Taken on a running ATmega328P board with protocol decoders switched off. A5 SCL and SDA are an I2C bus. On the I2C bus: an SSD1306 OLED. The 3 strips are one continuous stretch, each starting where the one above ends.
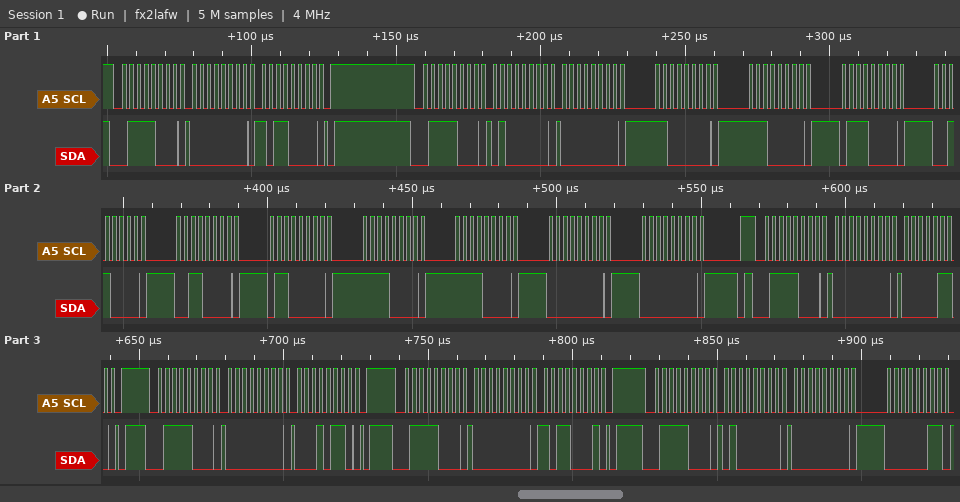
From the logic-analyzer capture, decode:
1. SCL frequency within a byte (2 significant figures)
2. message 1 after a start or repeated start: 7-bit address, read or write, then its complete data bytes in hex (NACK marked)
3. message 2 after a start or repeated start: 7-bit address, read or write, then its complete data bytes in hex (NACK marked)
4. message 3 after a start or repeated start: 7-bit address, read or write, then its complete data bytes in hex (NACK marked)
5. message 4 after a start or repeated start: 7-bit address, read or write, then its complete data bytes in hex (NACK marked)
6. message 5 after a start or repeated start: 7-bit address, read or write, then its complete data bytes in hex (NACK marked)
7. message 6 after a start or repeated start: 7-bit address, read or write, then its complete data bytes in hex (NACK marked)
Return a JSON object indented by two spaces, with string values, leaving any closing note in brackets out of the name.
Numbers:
{
  "SCL frequency within a byte": "400 kHz",
  "message 1 after a start or repeated start: 7-bit address, read or write, then its complete data bytes in hex": "0x3C write: 00 B0",
  "message 2 after a start or repeated start: 7-bit address, read or write, then its complete data bytes in hex": "0x3C write: 40 00 C0 E0 70 30 30 60 F0 F0 00 00",
  "message 3 after a start or repeated start: 7-bit address, read or write, then its complete data bytes in hex": "0x3C write: 00 06",
  "message 4 after a start or repeated start: 7-bit address, read or write, then its complete data bytes in hex": "0x3C write: 00 16",
  "message 5 after a start or repeated start: 7-bit address, read or write, then its complete data bytes in hex": "0x3C write: 00 B1",
  "message 6 after a start or repeated start: 7-bit address, read or write, then its complete data bytes in hex": "0x3C write: 40 00 03"
}
